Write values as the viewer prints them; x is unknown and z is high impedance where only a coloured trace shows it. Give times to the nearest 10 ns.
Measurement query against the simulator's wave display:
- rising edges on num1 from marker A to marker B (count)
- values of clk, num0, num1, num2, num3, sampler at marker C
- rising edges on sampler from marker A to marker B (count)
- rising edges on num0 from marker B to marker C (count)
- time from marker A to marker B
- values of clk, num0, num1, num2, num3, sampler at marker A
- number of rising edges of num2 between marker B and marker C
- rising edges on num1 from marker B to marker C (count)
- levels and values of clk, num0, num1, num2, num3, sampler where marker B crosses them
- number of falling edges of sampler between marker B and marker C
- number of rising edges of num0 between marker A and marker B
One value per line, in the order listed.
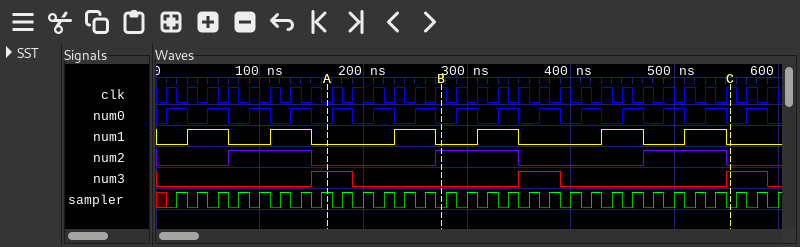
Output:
1
clk=1, num0=0, num1=0, num2=0, num3=1, sampler=0
5
7
110 ns
clk=0, num0=0, num1=0, num2=0, num3=1, sampler=1
1
3
clk=1, num0=0, num1=0, num2=1, num3=0, sampler=0
14
3
